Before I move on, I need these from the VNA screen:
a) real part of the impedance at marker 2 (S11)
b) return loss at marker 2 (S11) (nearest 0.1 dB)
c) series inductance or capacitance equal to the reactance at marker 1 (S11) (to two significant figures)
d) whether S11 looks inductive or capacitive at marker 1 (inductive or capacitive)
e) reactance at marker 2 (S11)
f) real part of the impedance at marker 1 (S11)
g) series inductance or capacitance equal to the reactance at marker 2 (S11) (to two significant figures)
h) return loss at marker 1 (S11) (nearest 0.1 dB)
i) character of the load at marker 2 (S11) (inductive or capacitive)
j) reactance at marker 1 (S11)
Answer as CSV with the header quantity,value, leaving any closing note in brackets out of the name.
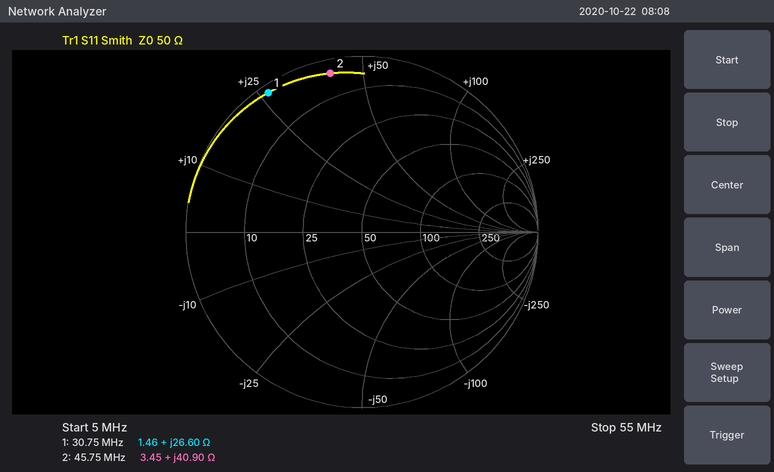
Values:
quantity,value
real part of the impedance at marker 2,3.45 Ω
return loss at marker 2 (S11),0.7 dB
series inductance or capacitance equal to the reactance at marker 1 (S11),140 nH
whether S11 looks inductive or capacitive at marker 1,inductive
reactance at marker 2,+40.90 Ω
real part of the impedance at marker 1,1.46 Ω
series inductance or capacitance equal to the reactance at marker 2 (S11),140 nH
return loss at marker 1 (S11),0.4 dB
character of the load at marker 2 (S11),inductive
reactance at marker 1,+26.60 Ω
